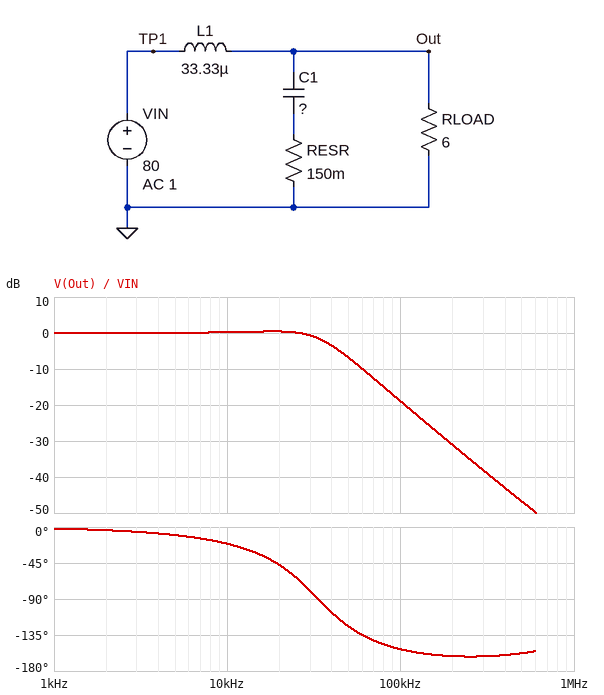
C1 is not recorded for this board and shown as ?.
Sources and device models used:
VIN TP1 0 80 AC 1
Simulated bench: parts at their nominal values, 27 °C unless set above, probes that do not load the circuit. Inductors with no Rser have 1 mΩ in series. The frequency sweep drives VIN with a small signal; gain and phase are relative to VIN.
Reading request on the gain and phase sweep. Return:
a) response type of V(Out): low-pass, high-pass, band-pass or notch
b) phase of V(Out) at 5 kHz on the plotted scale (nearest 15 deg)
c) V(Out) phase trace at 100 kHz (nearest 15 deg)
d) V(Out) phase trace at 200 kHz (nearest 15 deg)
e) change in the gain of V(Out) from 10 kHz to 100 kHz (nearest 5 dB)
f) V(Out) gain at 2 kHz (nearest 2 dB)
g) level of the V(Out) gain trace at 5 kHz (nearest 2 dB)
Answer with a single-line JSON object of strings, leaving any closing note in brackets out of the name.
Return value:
{"response type of V(Out): low-pass, high-pass, band-pass or notch": "low-pass", "phase of V(Out) at 5 kHz on the plotted scale": "-15 deg", "V(Out) phase trace at 100 kHz": "-150 deg", "V(Out) phase trace at 200 kHz": "-165 deg", "change in the gain of V(Out) from 10 kHz to 100 kHz": "-20 dB", "V(Out) gain at 2 kHz": "0 dB", "level of the V(Out) gain trace at 5 kHz": "0 dB"}
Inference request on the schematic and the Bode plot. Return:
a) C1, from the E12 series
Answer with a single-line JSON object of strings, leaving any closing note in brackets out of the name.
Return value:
{"C1, from the E12 series": "680 nF"}
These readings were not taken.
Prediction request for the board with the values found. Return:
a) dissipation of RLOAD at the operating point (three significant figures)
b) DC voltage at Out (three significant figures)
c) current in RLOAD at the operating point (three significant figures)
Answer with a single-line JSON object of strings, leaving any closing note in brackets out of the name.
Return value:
{"dissipation of RLOAD at the operating point": "1.07 kW", "DC voltage at Out": "80.0 V", "current in RLOAD at the operating point": "13.3 A"}
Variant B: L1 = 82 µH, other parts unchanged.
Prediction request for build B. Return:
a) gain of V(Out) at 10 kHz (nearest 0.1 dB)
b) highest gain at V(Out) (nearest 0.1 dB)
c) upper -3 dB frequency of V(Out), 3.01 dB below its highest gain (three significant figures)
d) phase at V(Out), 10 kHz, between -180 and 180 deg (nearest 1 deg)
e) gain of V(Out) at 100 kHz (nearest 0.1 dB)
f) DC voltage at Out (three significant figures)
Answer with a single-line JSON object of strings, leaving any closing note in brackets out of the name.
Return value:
{"gain of V(Out) at 10 kHz": "-1.3 dB", "highest gain at V(Out)": "0 dB", "upper -3 dB frequency of V(Out), 3.01 dB below its highest gain": "15.5 kHz", "phase at V(Out), 10 kHz, between -180 and 180 deg": "-48 deg", "gain of V(Out) at 100 kHz": "-27.3 dB", "DC voltage at Out": "80.0 V"}
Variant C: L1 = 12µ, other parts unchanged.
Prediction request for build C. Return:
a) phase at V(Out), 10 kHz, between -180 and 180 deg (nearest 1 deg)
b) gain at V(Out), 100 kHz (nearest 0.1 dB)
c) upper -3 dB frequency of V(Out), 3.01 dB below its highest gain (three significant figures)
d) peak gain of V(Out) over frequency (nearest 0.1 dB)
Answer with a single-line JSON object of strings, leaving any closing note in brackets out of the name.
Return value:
{"phase at V(Out), 10 kHz, between -180 and 180 deg": "-7 deg", "gain at V(Out), 100 kHz": "-8.5 dB", "upper -3 dB frequency of V(Out), 3.01 dB below its highest gain": "65.4 kHz", "peak gain of V(Out) over frequency": "3.4 dB"}
